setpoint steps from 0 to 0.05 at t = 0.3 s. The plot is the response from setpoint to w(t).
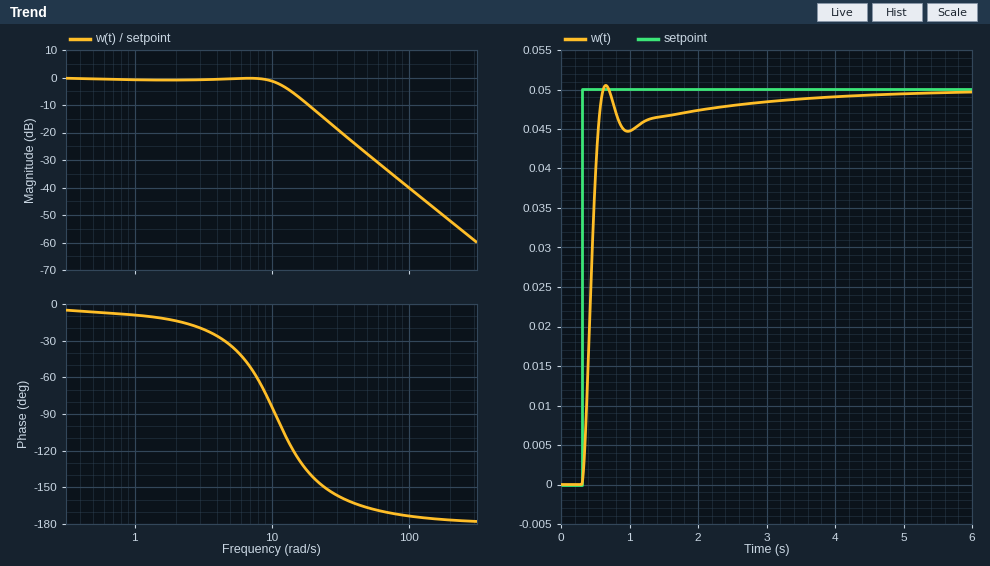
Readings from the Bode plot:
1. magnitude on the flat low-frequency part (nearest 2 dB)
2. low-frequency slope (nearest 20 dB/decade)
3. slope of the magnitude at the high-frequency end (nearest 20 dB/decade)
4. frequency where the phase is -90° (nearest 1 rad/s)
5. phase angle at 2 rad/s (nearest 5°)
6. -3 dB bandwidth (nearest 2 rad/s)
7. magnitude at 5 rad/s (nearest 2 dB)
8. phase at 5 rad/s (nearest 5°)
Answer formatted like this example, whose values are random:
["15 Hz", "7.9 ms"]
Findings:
["0 dB", "0 dB/decade", "-40 dB/decade", "11 rad/s", "-15°", "12 rad/s", "0 dB", "-35°"]
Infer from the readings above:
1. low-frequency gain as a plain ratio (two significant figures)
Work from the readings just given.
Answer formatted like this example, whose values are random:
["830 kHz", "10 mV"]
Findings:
["1.0"]
